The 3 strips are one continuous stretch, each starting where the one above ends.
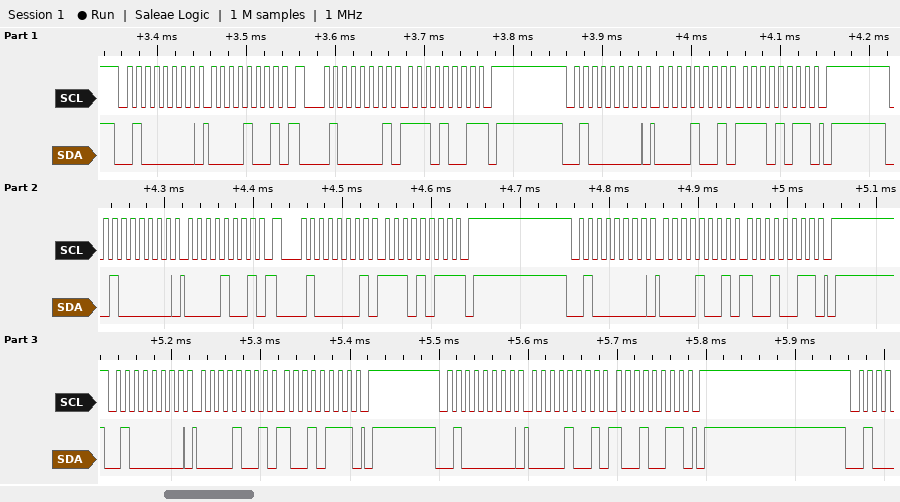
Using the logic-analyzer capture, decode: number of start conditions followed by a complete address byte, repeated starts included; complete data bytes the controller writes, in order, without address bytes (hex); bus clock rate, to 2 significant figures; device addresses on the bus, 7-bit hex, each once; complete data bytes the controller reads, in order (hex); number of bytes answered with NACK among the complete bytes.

8
09 09 EB 09 09 93 09 97 09 93
100 kHz
0x20
E9 EB
2
